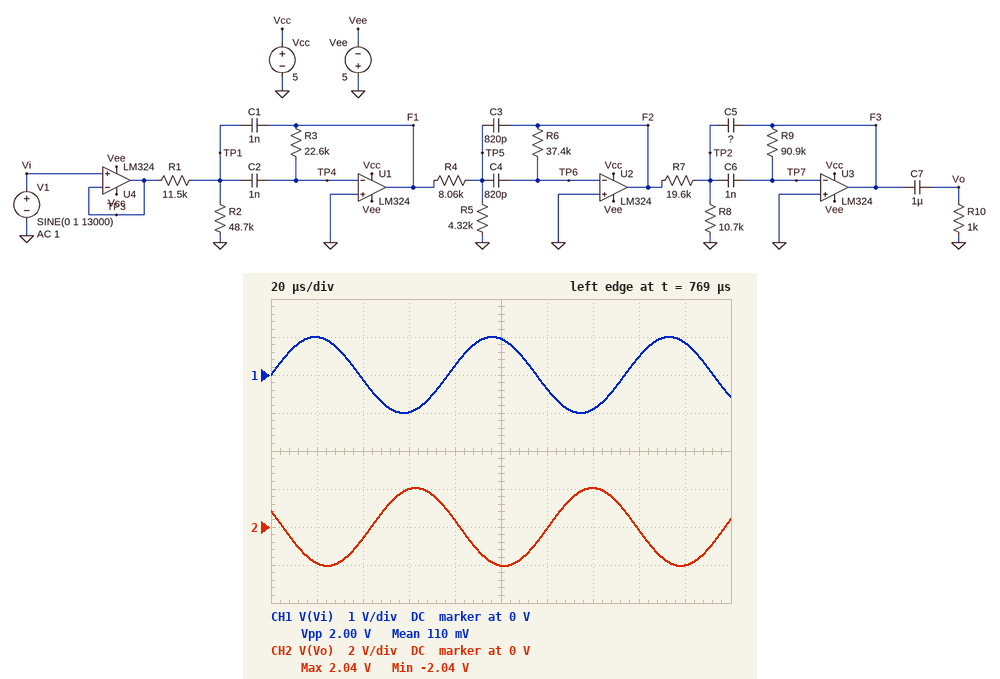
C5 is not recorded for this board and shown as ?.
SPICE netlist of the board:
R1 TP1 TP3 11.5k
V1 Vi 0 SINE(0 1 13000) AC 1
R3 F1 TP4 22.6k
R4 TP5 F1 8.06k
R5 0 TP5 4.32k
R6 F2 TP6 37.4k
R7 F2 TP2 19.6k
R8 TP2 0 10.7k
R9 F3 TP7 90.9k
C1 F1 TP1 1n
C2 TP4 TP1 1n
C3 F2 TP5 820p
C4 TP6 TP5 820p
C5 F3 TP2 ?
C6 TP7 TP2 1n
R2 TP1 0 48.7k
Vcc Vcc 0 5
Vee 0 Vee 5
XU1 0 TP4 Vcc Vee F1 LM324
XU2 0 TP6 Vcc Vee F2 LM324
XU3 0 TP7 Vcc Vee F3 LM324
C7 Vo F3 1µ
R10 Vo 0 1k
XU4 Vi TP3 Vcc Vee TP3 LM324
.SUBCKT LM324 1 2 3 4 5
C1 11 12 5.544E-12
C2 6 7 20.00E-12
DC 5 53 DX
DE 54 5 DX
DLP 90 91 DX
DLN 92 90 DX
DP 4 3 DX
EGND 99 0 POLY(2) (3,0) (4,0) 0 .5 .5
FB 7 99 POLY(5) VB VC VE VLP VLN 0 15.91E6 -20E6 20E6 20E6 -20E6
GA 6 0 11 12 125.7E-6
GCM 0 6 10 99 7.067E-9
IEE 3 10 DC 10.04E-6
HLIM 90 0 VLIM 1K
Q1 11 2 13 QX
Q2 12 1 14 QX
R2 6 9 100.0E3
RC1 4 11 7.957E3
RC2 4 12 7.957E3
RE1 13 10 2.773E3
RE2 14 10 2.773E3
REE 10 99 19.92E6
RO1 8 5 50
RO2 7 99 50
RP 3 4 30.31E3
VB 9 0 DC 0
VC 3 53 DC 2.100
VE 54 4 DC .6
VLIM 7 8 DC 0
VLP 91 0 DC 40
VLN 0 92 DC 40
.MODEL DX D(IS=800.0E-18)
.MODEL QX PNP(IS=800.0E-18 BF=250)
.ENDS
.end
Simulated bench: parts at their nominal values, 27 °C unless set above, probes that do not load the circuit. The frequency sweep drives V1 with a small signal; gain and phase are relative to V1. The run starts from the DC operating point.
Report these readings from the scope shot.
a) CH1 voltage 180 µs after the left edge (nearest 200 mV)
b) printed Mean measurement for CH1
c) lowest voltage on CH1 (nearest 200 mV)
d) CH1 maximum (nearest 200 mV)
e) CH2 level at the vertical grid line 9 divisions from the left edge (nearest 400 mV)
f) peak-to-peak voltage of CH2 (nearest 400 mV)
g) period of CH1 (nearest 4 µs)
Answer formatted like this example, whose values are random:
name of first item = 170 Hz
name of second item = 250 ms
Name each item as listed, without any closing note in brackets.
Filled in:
CH1 voltage 180 µs after the left edge = 800 mV
printed Mean measurement for CH1 = 110 mV
lowest voltage on CH1 = -1.0 V
CH1 maximum = 1.0 V
CH2 level at the vertical grid line 9 divisions from the left edge = -2.0 V
peak-to-peak voltage of CH2 = 4.0 V
period of CH1 = 76 µs
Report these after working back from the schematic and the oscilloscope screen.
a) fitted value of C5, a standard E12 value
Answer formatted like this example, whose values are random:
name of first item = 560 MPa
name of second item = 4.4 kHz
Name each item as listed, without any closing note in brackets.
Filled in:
fitted value of C5, a standard E12 value = 560 pF
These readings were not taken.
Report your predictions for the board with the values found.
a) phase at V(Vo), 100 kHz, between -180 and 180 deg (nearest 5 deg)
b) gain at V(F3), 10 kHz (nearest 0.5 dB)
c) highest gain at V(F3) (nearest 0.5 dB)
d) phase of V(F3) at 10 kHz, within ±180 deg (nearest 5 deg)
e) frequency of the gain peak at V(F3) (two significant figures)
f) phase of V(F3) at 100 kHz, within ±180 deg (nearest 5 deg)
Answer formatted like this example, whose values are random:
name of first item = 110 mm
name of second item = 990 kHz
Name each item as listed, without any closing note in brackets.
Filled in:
phase at V(Vo), 100 kHz, between -180 and 180 deg = -95 deg
gain at V(F3), 10 kHz = 6.5 dB
highest gain at V(F3) = 6.5 dB
phase of V(F3) at 10 kHz, within ±180 deg = -140 deg
frequency of the gain peak at V(F3) = 10 kHz
phase of V(F3) at 100 kHz, within ±180 deg = -95 deg
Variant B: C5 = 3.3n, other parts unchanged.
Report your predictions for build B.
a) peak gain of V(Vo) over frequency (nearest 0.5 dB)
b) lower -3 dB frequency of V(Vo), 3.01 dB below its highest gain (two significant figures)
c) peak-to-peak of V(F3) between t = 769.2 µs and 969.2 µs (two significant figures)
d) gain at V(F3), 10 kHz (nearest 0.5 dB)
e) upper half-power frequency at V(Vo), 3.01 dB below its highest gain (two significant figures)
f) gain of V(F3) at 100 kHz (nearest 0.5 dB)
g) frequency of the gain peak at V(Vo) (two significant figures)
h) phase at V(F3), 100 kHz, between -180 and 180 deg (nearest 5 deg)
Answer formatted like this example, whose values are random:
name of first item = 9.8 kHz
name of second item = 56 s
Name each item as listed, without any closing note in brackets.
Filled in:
peak gain of V(Vo) over frequency = -11.0 dB
lower -3 dB frequency of V(Vo), 3.01 dB below its highest gain = 7.7 kHz
peak-to-peak of V(F3) between t = 769.2 µs and 969.2 µs = 530 mV
gain at V(F3), 10 kHz = -12.5 dB
upper half-power frequency at V(Vo), 3.01 dB below its highest gain = 20 kHz
gain of V(F3) at 100 kHz = -62.0 dB
frequency of the gain peak at V(Vo) = 15 kHz
phase at V(F3), 100 kHz, between -180 and 180 deg = -100 deg
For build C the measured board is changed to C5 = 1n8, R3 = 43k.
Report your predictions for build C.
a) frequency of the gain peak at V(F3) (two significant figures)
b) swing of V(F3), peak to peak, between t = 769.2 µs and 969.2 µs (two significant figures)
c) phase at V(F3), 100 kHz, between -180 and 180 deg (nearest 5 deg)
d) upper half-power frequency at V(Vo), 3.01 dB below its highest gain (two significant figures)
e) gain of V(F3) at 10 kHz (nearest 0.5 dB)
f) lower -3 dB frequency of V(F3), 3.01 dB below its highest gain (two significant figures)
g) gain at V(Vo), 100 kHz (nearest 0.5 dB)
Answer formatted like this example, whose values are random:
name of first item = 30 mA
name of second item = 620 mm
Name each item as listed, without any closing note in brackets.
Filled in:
frequency of the gain peak at V(F3) = 7.1 kHz
swing of V(F3), peak to peak, between t = 769.2 µs and 969.2 µs = 1.3 V
phase at V(F3), 100 kHz, between -180 and 180 deg = -100 deg
upper half-power frequency at V(Vo), 3.01 dB below its highest gain = 14 kHz
gain of V(F3) at 10 kHz = -2.0 dB
lower -3 dB frequency of V(F3), 3.01 dB below its highest gain = 4.6 kHz
gain at V(Vo), 100 kHz = -57.0 dB
